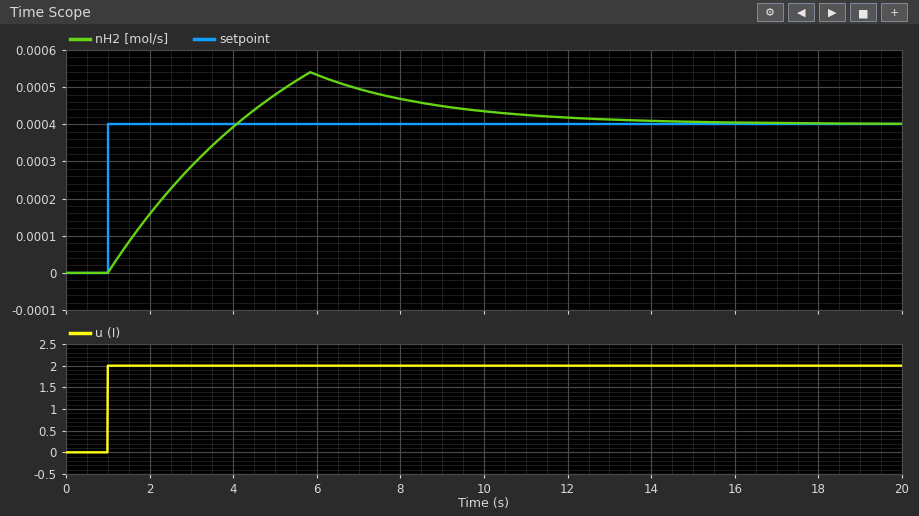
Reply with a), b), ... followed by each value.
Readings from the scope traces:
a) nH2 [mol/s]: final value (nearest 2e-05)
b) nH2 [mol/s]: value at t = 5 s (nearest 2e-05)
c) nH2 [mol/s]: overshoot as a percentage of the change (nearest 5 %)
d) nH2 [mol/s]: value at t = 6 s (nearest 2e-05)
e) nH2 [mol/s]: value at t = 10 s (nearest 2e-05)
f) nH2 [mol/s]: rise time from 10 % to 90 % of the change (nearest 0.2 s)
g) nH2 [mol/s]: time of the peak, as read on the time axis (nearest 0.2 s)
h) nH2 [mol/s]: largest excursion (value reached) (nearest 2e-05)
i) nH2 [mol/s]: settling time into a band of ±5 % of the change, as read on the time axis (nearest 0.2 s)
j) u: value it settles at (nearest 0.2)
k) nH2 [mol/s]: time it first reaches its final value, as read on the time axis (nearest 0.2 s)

a) 0.00040
b) 0.00048
c) 35 %
d) 0.00054
e) 0.00044
f) 2.4 s
g) 5.8 s
h) 0.00054
i) 11.6 s
j) 2.0
k) 4.0 s
